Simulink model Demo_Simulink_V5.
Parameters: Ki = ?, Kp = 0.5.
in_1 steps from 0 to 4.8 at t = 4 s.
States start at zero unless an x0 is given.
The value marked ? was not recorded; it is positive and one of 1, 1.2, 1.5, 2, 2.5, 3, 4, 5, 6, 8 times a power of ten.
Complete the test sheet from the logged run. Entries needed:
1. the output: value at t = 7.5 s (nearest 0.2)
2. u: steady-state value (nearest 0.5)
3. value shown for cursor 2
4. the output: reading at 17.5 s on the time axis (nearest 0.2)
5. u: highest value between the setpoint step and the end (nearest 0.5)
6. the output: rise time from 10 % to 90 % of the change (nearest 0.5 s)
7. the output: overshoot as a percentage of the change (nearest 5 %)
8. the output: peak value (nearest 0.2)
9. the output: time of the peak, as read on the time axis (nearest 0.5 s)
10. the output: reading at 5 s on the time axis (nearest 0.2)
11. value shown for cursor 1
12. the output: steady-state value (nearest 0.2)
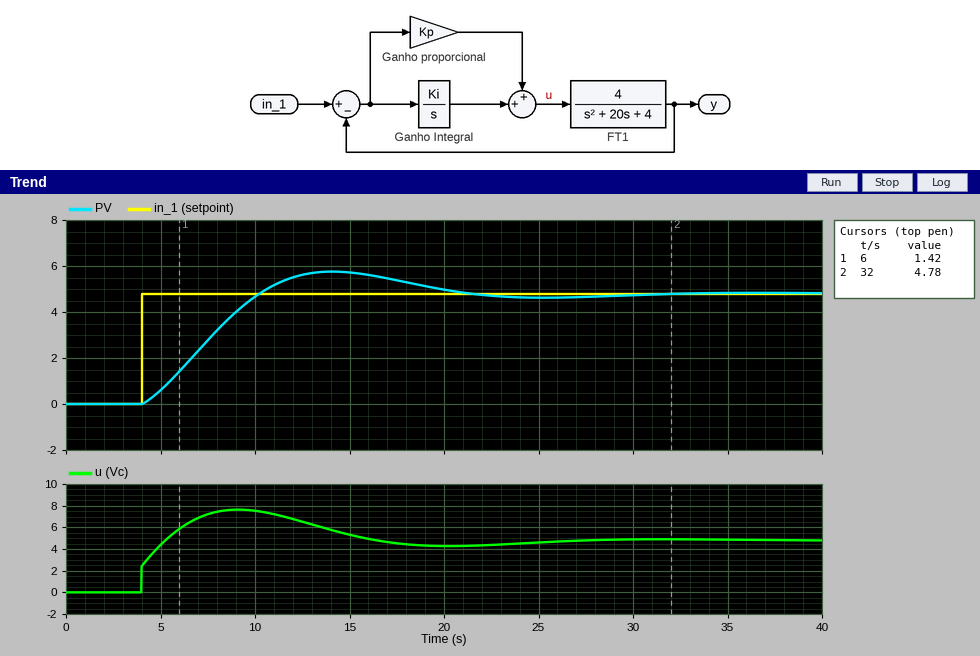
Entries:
2.8
5.0
4.78
5.4
7.5
4.5 s
20 %
5.8
14.0 s
0.6
1.42
4.8
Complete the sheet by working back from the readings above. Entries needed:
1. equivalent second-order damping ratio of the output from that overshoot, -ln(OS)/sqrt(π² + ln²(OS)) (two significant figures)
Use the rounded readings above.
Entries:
0.46
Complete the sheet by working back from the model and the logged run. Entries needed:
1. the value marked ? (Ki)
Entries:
0.5
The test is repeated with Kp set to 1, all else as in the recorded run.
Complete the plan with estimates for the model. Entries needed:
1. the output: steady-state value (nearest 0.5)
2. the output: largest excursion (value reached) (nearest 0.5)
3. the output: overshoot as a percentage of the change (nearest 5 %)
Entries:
5.0
5.5
10 %
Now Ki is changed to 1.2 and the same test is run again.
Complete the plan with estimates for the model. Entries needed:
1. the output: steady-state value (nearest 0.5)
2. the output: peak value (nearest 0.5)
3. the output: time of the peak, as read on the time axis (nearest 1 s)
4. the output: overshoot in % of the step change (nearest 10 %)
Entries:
5.0
6.5
10 s
40 %
